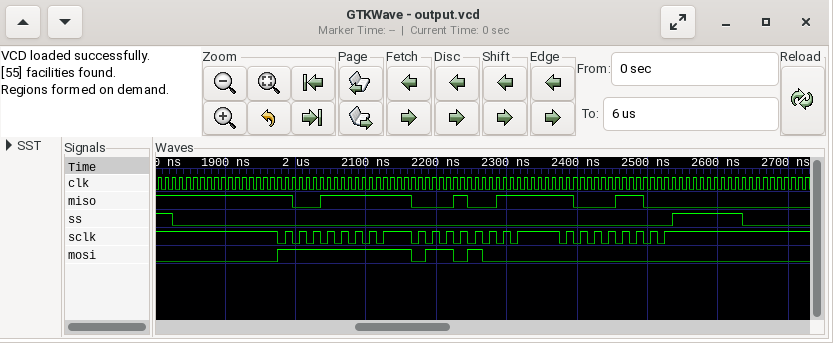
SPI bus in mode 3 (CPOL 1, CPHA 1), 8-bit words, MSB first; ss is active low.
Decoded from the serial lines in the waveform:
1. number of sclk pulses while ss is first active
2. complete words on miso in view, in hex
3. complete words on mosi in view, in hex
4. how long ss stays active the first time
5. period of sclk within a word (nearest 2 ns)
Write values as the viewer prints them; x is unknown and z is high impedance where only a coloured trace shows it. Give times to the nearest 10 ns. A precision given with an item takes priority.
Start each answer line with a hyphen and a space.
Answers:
- 24
- 9F, 13, 8C
- FF, 68, 00
- 710 ns
- 20 ns
